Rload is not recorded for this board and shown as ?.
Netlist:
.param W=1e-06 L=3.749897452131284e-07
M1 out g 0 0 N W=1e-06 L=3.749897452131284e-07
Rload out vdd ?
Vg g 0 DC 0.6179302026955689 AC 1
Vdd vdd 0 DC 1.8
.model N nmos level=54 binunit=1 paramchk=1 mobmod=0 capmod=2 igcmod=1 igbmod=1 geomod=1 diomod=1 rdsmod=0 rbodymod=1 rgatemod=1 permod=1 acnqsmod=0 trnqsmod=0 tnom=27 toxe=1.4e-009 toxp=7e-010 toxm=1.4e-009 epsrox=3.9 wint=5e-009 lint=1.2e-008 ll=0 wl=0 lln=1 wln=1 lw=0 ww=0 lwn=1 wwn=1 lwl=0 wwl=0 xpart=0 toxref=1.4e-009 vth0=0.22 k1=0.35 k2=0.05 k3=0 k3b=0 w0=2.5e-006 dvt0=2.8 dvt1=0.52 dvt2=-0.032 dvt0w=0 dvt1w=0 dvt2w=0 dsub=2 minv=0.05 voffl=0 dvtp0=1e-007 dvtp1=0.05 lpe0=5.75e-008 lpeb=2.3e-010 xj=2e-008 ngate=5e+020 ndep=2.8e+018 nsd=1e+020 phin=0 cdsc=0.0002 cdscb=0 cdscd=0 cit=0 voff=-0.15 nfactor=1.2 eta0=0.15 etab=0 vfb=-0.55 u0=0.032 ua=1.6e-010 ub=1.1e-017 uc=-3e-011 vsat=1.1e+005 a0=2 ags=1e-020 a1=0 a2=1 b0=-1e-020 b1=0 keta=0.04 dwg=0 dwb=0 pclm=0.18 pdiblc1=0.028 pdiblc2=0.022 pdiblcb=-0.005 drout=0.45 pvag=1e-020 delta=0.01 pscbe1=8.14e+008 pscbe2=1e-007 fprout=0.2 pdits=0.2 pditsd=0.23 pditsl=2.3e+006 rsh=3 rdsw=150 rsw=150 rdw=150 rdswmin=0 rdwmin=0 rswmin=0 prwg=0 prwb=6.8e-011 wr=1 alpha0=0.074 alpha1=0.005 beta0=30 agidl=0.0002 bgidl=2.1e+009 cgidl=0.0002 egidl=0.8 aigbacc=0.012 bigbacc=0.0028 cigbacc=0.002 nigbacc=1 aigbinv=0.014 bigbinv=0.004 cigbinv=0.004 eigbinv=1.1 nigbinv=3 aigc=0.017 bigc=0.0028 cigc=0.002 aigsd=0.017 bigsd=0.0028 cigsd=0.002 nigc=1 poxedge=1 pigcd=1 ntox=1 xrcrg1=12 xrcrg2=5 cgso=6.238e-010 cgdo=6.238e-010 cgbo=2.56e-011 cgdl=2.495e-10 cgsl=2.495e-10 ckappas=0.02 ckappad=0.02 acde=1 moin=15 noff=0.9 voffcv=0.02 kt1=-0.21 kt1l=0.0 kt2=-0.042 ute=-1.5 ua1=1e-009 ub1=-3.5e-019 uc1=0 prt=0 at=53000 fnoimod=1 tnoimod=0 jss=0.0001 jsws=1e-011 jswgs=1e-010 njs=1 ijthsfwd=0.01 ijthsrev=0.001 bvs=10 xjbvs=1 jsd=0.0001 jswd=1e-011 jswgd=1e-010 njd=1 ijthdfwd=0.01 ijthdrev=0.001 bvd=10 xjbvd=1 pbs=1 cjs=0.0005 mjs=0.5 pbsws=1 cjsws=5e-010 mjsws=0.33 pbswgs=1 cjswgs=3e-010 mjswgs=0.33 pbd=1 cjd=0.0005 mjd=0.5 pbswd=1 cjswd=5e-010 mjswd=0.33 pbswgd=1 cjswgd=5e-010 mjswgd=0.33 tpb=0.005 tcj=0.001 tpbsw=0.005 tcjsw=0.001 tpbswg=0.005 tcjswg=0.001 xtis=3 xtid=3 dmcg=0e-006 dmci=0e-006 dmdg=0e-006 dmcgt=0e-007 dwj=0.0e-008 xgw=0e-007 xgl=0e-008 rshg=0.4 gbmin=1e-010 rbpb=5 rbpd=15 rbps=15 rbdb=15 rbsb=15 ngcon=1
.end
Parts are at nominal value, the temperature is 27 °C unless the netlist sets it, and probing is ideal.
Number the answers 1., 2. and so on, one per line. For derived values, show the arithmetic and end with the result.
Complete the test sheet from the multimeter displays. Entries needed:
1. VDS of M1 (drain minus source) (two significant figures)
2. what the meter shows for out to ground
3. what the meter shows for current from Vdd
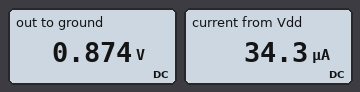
1. 874 mV = 870 mV
2. 0.874 V
3. 34.3 µA
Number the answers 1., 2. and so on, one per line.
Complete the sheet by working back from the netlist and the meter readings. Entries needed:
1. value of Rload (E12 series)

1. 27 kΩ
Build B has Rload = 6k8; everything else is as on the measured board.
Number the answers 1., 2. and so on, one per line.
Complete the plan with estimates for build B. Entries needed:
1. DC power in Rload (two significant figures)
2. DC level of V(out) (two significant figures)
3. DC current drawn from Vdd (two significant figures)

1. 9.8 µW
2. 1.5 V
3. 38 µA
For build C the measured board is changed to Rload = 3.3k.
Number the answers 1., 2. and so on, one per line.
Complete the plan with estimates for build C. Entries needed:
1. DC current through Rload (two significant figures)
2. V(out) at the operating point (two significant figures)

1. 39 µA
2. 1.7 V
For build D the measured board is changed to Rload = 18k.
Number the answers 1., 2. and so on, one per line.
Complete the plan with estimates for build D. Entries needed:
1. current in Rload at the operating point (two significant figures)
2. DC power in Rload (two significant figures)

1. 36 µA
2. 23 µW
